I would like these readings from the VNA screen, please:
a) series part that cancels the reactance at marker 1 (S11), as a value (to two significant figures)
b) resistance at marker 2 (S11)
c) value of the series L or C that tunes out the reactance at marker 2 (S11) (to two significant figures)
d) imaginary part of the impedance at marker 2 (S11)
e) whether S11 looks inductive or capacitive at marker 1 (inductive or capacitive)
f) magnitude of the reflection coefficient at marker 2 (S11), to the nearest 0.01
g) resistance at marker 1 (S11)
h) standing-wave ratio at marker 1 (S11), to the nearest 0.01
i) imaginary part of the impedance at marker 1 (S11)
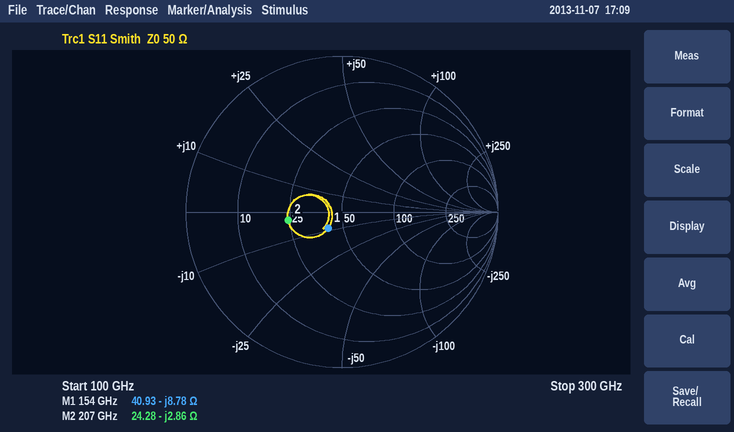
9.1 pH
24.28 Ω
2.2 pH
-2.86 Ω
capacitive
0.35
40.93 Ω
1.32
-8.78 Ω
